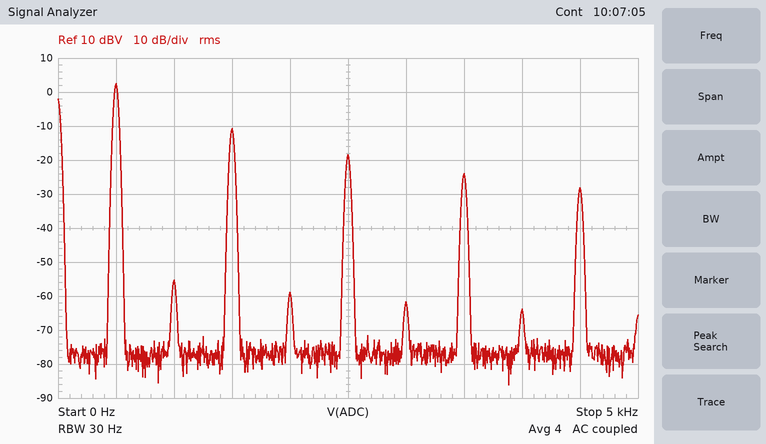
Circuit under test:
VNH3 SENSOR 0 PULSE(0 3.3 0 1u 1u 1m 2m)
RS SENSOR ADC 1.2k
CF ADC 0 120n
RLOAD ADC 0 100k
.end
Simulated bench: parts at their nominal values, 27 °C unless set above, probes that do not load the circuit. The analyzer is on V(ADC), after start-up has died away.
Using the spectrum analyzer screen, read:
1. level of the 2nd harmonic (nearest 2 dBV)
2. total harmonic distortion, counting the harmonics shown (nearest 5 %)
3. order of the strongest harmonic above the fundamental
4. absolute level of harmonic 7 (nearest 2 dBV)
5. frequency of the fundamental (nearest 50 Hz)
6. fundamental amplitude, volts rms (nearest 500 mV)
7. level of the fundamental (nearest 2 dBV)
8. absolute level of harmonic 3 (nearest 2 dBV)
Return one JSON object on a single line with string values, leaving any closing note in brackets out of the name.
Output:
{"level of the 2nd harmonic": "-56 dBV", "total harmonic distortion, counting the harmonics shown": "25 %", "order of the strongest harmonic above the fundamental": "3", "absolute level of harmonic 7": "-24 dBV", "frequency of the fundamental": "500 Hz", "fundamental amplitude, volts rms": "1.5 V", "level of the fundamental": "2 dBV", "absolute level of harmonic 3": "-10 dBV"}
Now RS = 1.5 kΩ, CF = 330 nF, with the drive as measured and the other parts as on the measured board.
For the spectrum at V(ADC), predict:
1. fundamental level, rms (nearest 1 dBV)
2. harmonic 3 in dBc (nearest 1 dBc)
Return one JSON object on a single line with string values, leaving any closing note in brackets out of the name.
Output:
{"fundamental level, rms": "-2 dBV", "harmonic 3 in dBc": "-18 dBc"}
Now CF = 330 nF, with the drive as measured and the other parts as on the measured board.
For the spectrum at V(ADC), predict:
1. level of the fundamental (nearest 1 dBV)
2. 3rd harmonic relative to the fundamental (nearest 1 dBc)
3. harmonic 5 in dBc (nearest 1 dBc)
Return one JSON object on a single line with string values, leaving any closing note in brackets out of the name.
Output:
{"level of the fundamental": "-1 dBV", "3rd harmonic relative to the fundamental": "-17 dBc", "harmonic 5 in dBc": "-26 dBc"}
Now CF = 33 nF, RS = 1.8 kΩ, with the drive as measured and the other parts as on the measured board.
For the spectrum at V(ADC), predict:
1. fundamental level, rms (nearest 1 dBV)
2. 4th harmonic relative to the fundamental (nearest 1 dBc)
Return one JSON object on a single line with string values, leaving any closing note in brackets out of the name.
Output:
{"fundamental level, rms": "3 dBV", "4th harmonic relative to the fundamental": "-58 dBc"}
